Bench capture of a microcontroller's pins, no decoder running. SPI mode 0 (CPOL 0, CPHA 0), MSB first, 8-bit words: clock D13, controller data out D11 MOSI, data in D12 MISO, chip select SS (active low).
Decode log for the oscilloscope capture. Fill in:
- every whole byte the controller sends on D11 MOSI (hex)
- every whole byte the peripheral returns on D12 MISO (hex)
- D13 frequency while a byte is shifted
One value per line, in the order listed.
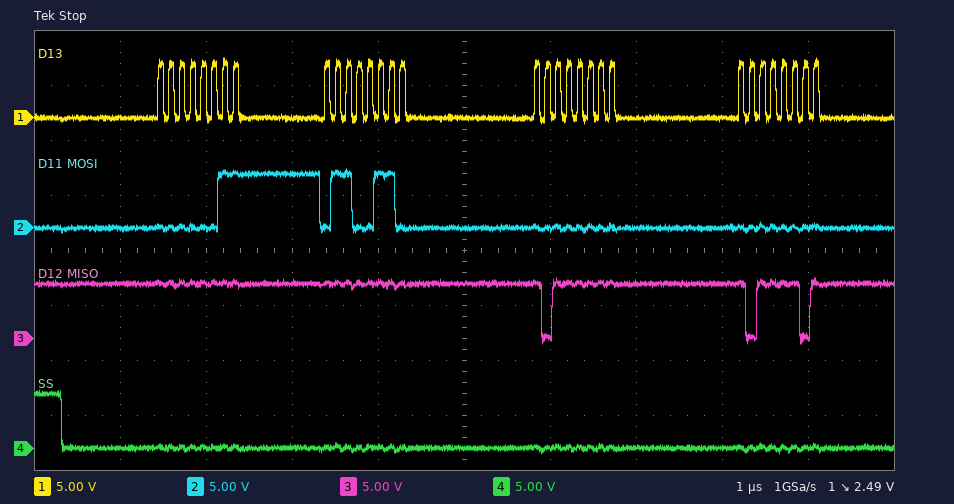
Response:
03 66 00 00
FF FF BF BD
8 MHz
